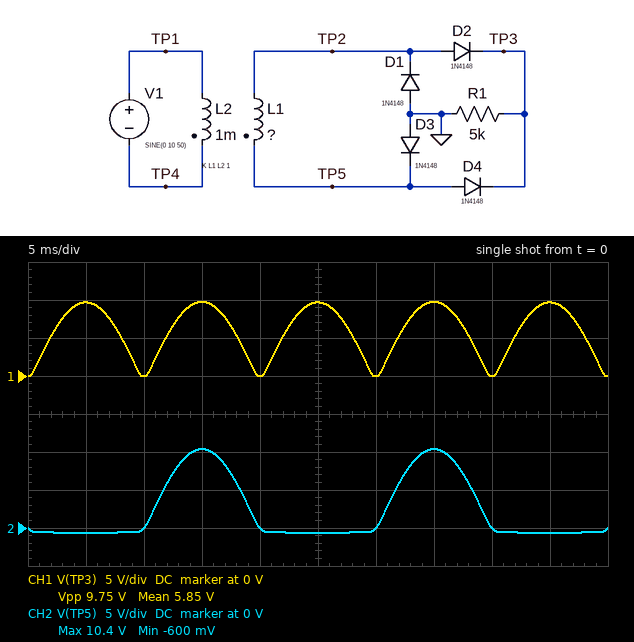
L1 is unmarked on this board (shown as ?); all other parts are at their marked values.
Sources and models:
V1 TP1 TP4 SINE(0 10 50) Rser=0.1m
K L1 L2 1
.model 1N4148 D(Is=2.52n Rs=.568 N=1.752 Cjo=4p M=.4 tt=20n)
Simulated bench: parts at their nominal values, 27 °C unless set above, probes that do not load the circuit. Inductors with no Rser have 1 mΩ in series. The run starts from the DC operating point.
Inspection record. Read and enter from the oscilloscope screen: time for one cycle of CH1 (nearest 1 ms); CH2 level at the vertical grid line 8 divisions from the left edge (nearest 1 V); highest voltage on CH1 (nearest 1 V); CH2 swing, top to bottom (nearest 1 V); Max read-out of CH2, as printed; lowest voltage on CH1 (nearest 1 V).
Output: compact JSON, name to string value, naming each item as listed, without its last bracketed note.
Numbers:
{"time for one cycle of CH1": "10 ms", "CH2 level at the vertical grid line 8 divisions from the left edge": "0 V", "highest voltage on CH1": "10 V", "CH2 swing, top to bottom": "11 V", "Max read-out of CH2, as printed": "10.4 V", "lowest voltage on CH1": "0 V"}
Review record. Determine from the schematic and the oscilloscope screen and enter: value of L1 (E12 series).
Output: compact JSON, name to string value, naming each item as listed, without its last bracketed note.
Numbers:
{"value of L1": "1.2 mH"}
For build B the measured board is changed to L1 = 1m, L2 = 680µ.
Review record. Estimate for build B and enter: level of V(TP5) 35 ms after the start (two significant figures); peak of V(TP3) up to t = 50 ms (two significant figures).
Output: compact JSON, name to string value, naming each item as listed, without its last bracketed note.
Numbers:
{"level of V(TP5) 35 ms after the start": "12 V", "peak of V(TP3) up to t = 50 ms": "11 V"}
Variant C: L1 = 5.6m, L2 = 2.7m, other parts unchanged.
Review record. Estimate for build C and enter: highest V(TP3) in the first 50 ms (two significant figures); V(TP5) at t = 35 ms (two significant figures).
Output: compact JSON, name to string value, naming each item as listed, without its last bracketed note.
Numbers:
{"highest V(TP3) in the first 50 ms": "13 V", "V(TP5) at t = 35 ms": "14 V"}
